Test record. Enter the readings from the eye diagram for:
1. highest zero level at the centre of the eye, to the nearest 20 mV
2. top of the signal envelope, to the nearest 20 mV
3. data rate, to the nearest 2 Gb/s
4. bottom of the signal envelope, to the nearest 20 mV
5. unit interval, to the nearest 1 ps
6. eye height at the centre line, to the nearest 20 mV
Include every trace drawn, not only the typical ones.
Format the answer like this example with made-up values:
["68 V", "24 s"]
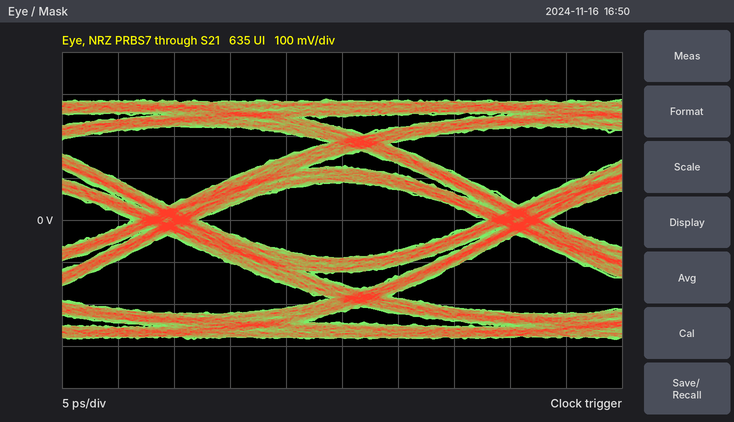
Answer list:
["-100 mV", "280 mV", "32 Gb/s", "-280 mV", "31 ps", "180 mV"]
